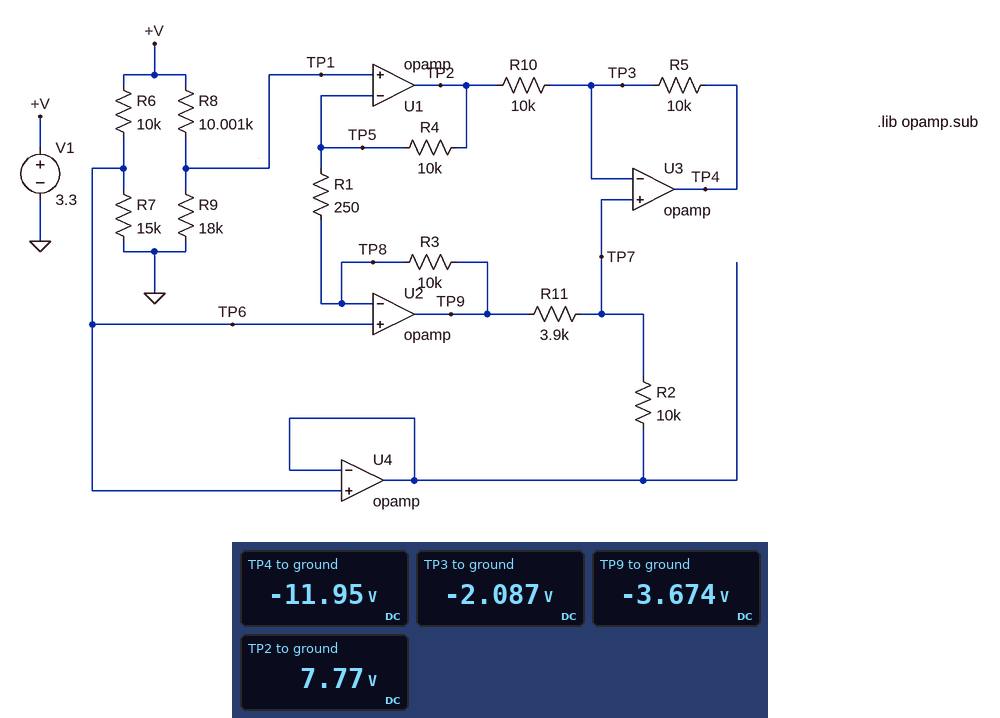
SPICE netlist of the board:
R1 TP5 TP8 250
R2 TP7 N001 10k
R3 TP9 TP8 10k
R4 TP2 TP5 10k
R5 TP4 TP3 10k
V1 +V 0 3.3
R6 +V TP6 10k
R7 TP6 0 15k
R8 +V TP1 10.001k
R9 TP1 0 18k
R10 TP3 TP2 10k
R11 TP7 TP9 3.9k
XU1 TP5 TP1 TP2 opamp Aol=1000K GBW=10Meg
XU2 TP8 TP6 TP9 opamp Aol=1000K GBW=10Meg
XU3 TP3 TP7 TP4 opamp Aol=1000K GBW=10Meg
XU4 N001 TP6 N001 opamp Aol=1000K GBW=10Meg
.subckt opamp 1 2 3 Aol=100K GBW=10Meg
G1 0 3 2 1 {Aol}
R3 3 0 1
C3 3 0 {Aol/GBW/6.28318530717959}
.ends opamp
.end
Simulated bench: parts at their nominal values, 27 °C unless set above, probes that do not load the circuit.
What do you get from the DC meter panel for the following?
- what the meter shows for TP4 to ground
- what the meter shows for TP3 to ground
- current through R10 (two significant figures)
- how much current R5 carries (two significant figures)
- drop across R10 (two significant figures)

-11.95 V
-2.087 V
990 µA
990 µA
9.9 V
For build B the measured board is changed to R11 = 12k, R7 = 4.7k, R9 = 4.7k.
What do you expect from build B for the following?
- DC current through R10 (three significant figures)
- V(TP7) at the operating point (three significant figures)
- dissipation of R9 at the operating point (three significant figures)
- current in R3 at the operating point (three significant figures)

425 nA
1.06 V
237 µW
287 nA
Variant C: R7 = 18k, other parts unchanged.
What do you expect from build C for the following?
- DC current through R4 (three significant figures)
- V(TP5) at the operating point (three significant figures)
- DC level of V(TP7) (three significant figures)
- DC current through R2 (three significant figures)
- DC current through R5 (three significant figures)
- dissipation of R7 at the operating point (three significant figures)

303 nA
2.12 V
2.12 V
218 nA
528 nA
250 µW
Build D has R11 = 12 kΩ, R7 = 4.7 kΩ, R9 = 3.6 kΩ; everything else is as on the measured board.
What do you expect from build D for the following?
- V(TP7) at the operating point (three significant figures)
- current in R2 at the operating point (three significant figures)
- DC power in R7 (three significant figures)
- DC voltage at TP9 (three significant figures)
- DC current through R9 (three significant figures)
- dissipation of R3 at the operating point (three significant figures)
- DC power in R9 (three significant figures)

4.36 V
330 µA
237 µW
8.32 V
243 µA
5.28 mW
212 µW
